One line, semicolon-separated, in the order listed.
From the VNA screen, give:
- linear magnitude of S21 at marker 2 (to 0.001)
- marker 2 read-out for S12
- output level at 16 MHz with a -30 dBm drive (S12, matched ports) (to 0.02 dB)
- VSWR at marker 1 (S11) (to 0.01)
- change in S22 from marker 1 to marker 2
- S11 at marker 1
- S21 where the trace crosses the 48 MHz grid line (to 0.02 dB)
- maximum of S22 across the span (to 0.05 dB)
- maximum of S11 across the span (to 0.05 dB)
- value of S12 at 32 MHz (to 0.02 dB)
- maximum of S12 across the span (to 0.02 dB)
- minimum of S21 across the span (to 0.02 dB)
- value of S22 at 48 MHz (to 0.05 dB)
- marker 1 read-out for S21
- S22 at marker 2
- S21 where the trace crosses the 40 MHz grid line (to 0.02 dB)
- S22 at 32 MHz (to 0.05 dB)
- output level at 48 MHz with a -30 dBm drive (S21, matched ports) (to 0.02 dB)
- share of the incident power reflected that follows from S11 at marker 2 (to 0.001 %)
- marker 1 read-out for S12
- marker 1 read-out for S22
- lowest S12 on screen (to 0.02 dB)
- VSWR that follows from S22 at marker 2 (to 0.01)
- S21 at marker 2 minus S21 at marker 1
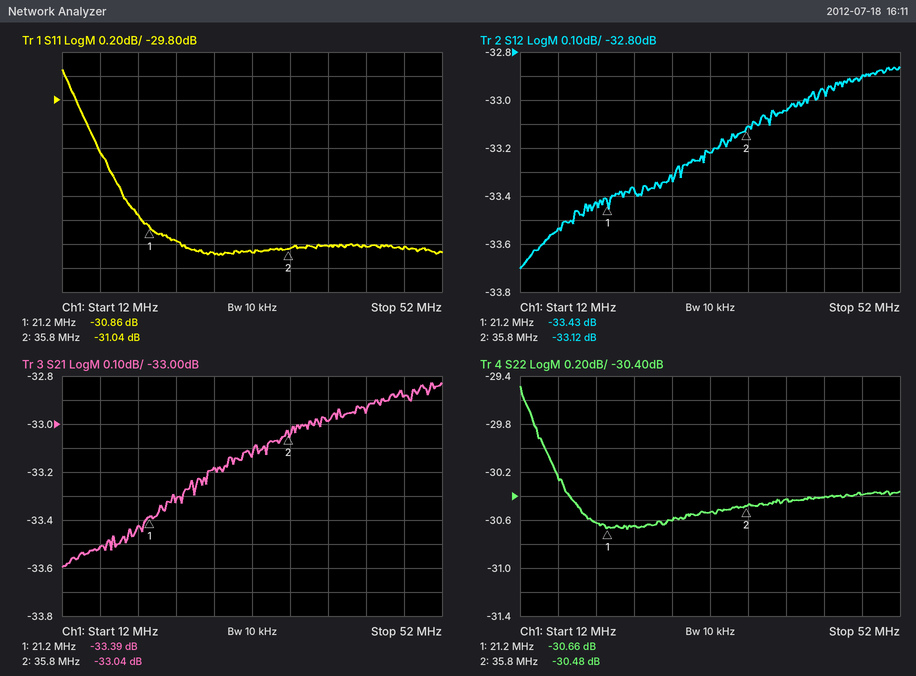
0.022; -33.12 dB; -63.54 dBm; 1.06; 0.18 dB; -30.86 dB; -32.88 dB; -29.50 dB; -29.55 dB; -33.22 dB; -32.86 dB; -33.60 dB; -30.40 dB; -33.39 dB; -30.48 dB; -32.98 dB; -30.55 dB; -62.88 dBm; 0.079 %; -33.43 dB; -30.66 dB; -33.70 dB; 1.06; 0.35 dB
